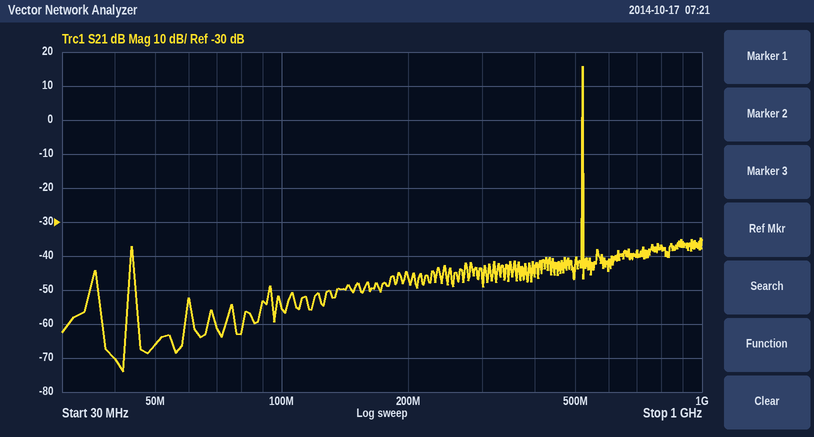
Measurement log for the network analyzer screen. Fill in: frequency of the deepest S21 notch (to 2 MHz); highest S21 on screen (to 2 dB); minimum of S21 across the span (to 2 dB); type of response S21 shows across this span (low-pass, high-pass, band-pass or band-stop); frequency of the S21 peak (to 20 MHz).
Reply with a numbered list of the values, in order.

1. 42 MHz
2. 16 dB
3. -74 dB
4. band-pass
5. 520 MHz
